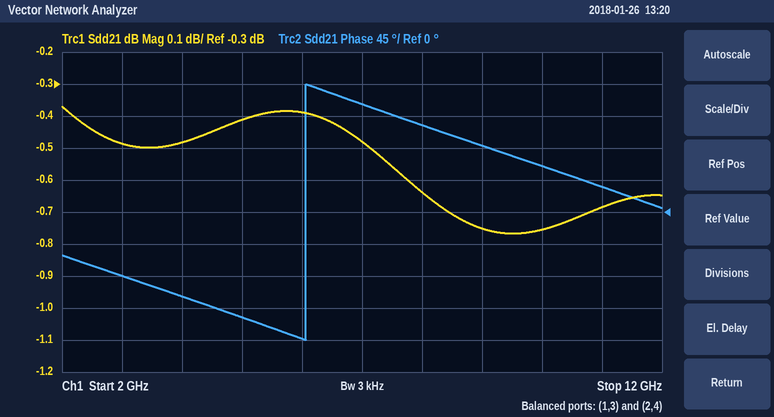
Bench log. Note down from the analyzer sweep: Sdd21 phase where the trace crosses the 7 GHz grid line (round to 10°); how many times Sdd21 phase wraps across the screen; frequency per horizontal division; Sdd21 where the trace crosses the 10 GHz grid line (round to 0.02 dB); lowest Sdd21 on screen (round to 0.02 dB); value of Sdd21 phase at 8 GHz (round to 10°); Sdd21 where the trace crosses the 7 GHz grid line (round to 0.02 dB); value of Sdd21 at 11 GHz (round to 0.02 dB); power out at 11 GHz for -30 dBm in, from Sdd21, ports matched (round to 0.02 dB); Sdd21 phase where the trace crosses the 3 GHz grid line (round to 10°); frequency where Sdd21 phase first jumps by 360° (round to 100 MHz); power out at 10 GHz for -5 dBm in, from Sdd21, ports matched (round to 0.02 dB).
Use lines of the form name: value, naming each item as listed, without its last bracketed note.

Sdd21 phase where the trace crosses the 7 GHz grid line: 150°
how many times Sdd21 phase wraps across the screen: 1
frequency per horizontal division: 1 GHz
Sdd21 where the trace crosses the 10 GHz grid line: -0.76 dB
lowest Sdd21 on screen: -0.76 dB
value of Sdd21 phase at 8 GHz: 120°
Sdd21 where the trace crosses the 7 GHz grid line: -0.48 dB
value of Sdd21 at 11 GHz: -0.68 dB
power out at 11 GHz for -30 dBm in, from Sdd21, ports matched: -30.68 dBm
Sdd21 phase where the trace crosses the 3 GHz grid line: -90°
frequency where Sdd21 phase first jumps by 360°: 6.1 GHz
power out at 10 GHz for -5 dBm in, from Sdd21, ports matched: -5.76 dBm
